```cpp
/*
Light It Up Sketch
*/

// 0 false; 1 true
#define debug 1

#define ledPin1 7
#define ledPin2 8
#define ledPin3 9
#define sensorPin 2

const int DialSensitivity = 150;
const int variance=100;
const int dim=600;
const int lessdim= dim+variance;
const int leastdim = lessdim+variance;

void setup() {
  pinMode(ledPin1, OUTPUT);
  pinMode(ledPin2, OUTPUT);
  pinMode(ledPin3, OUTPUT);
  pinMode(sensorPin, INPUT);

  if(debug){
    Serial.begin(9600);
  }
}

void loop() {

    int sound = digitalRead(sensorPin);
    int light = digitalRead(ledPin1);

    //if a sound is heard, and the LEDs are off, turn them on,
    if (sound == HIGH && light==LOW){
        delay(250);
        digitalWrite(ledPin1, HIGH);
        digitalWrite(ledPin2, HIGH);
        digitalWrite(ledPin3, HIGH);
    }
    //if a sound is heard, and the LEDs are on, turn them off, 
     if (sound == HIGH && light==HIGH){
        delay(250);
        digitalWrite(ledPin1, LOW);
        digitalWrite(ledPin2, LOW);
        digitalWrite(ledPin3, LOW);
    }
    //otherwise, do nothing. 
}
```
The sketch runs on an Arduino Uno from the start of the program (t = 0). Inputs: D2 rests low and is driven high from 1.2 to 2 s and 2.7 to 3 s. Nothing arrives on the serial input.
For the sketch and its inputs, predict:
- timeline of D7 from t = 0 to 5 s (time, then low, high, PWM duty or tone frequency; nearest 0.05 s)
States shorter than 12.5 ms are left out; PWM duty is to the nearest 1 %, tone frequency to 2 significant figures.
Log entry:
0 s low; 1.45 s high; 1.7 s low; 1.95 s high; 2.2 s low; 2.95 s high; 3.2 s low
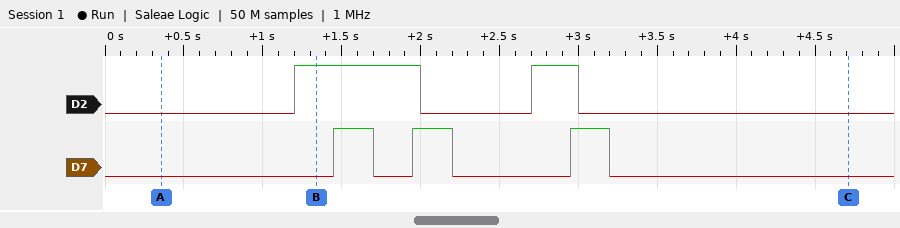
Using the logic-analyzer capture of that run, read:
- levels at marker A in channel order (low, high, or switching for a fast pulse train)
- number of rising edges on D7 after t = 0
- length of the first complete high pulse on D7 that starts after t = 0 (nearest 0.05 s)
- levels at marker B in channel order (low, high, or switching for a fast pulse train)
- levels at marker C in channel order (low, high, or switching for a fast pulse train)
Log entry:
D2 low, D7 low
3
0.25 s
D2 high, D7 low
D2 low, D7 low
